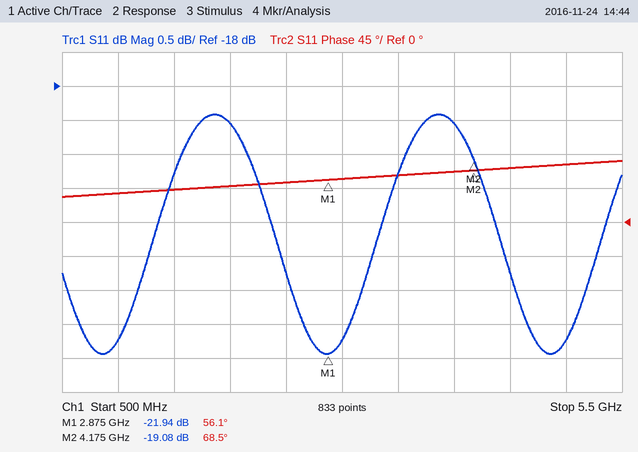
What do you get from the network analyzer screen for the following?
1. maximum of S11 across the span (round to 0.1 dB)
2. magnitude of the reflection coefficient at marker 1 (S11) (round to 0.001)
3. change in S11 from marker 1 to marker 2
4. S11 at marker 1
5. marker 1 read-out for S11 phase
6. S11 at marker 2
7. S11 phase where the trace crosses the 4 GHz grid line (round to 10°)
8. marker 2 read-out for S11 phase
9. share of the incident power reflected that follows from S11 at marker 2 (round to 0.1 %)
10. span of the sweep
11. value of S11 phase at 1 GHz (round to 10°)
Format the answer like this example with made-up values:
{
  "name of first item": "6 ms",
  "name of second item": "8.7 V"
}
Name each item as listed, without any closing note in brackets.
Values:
{
  "maximum of S11 across the span": "-18.4 dB",
  "magnitude of the reflection coefficient at marker 1 (S11)": "0.080",
  "change in S11 from marker 1 to marker 2": "2.86 dB",
  "S11 at marker 1": "-21.94 dB",
  "marker 1 read-out for S11 phase": "56.1°",
  "S11 at marker 2": "-19.08 dB",
  "S11 phase where the trace crosses the 4 GHz grid line": "70°",
  "marker 2 read-out for S11 phase": "68.5°",
  "share of the incident power reflected that follows from S11 at marker 2": "1.2 %",
  "span of the sweep": "5 GHz",
  "value of S11 phase at 1 GHz": "40°"
}
